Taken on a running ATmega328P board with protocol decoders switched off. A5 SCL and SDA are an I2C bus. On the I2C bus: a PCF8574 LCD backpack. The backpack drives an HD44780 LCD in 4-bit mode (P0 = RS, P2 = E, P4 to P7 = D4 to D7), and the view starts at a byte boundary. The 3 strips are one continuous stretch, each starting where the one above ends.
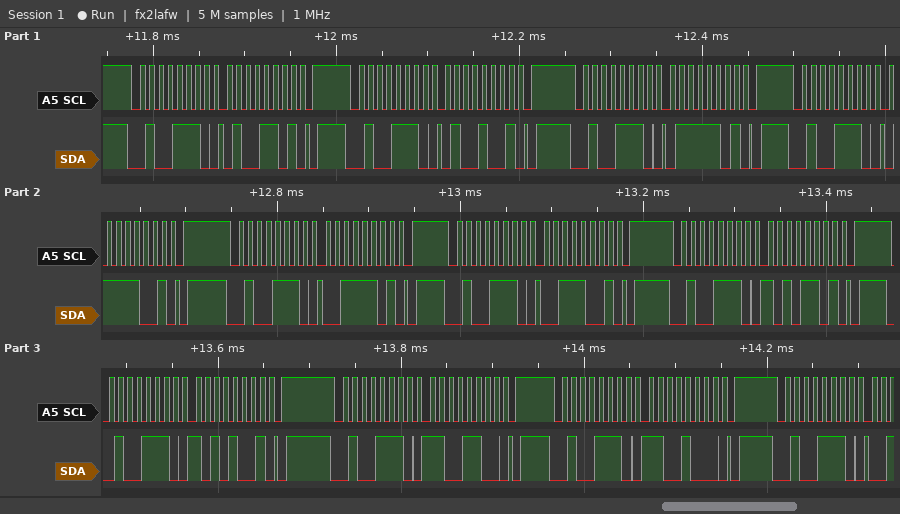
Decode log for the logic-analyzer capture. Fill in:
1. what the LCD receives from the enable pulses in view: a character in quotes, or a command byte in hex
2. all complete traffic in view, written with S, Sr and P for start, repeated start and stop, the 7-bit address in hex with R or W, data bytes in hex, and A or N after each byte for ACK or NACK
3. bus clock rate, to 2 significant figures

'G' ':'
S 27W A 4D A P S 27W A 49 A P S 27W A 7D A P S 27W A 79 A P S 27W A 3D A P S 27W A 39 A P S 27W A AD A P S 27W A A9 A P S 27W A CC A P S 27W A C8 A P S 27W A
100 kHz
